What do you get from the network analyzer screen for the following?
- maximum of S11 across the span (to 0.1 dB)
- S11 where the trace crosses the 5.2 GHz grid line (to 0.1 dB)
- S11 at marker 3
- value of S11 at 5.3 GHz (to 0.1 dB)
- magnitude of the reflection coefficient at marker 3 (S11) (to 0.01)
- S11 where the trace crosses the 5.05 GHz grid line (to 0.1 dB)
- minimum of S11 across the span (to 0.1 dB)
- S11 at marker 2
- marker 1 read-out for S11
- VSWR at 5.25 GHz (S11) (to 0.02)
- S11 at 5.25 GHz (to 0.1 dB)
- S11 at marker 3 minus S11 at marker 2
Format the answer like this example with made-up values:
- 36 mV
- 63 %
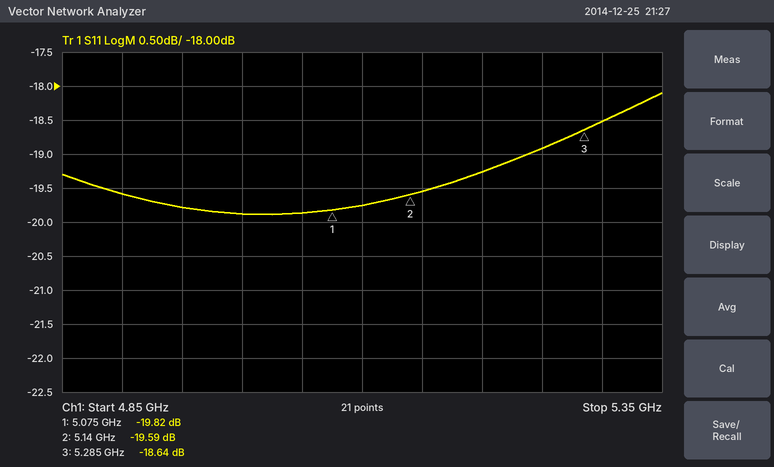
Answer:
- -18.1 dB
- -19.3 dB
- -18.64 dB
- -18.5 dB
- 0.12
- -19.9 dB
- -19.9 dB
- -19.59 dB
- -19.82 dB
- 1.26
- -18.9 dB
- 0.95 dB
